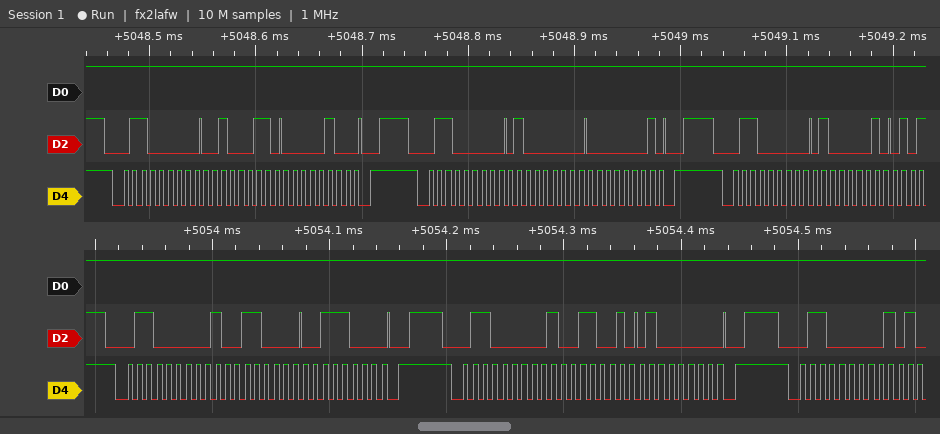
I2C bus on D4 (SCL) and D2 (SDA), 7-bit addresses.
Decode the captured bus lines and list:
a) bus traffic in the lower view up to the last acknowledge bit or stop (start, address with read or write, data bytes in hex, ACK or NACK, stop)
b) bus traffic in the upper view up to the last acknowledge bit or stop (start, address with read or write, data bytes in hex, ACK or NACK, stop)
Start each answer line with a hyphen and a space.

- start, address 30 write ACK, 98 ACK, 38 ACK, stop, start, address 30 write ACK, 99 ACK, 40 ACK, stop, start, address 30 write ACK
- start, address 30 write ACK, 23 ACK, 04 ACK, stop, start, address 30 write ACK, 40 ACK, 01 ACK, stop, start, address 30 write ACK, 41 ACK
